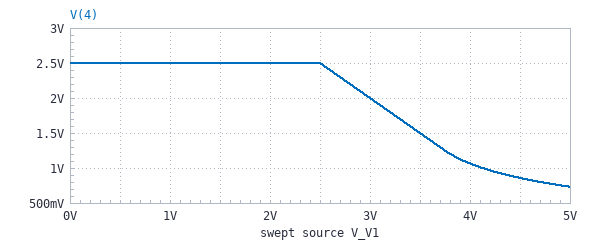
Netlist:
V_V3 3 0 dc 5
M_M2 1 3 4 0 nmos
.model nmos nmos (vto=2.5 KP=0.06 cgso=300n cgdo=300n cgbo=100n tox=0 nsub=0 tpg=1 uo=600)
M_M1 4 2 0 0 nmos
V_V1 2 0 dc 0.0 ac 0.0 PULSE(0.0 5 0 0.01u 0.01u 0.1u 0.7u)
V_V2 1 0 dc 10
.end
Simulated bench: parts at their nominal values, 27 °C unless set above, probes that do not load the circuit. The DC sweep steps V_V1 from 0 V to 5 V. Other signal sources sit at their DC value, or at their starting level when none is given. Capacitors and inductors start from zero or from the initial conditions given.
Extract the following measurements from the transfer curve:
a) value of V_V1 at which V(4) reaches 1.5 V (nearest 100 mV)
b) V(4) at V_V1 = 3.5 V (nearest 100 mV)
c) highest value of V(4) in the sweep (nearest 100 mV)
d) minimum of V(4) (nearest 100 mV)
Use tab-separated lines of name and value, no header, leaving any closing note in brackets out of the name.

value of V_V1 at which V(4) reaches 1.5 V	3.5 V
V(4) at V_V1 = 3.5 V	1.5 V
highest value of V(4) in the sweep	2.5 V
minimum of V(4)	700 mV
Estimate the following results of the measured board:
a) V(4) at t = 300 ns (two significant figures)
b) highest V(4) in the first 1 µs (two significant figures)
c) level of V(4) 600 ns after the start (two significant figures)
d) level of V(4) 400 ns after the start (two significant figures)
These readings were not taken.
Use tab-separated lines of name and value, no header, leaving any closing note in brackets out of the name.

V(4) at t = 300 ns	2.5 V
highest V(4) in the first 1 µs	4.0 V
level of V(4) 600 ns after the start	2.5 V
level of V(4) 400 ns after the start	2.5 V
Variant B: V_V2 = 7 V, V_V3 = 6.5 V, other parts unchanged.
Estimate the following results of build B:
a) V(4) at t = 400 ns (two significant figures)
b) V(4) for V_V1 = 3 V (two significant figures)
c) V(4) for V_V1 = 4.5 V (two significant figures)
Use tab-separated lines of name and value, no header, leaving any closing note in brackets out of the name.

V(4) at t = 400 ns	4.0 V
V(4) for V_V1 = 3 V	3.5 V
V(4) for V_V1 = 4.5 V	2.0 V
